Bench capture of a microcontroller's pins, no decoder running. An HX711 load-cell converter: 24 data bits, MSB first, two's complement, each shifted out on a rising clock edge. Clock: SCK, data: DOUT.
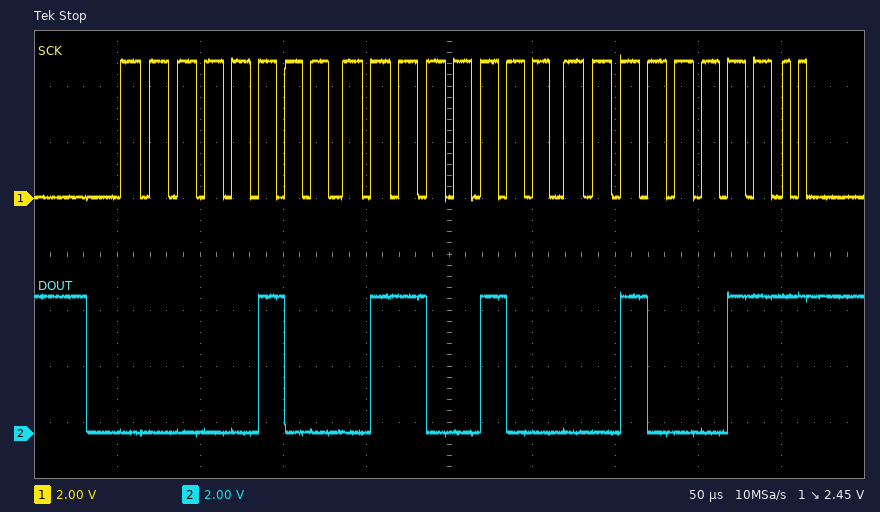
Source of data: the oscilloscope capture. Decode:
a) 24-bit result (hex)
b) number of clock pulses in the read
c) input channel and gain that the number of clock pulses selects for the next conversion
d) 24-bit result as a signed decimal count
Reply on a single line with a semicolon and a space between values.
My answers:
0x046423; 26; channel B, gain 32; 287779
